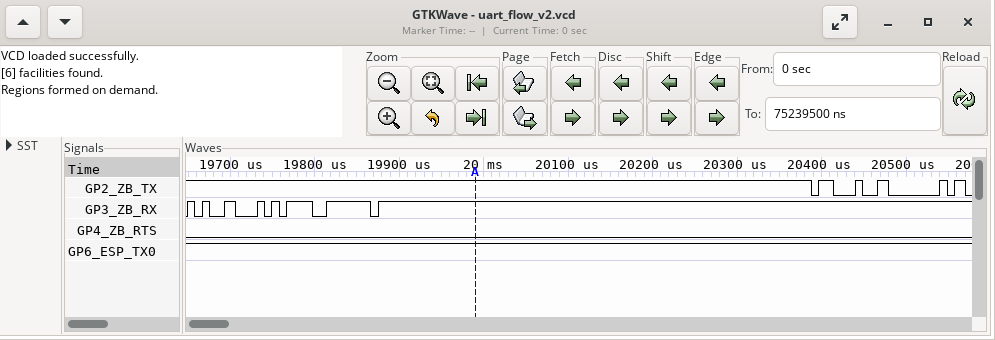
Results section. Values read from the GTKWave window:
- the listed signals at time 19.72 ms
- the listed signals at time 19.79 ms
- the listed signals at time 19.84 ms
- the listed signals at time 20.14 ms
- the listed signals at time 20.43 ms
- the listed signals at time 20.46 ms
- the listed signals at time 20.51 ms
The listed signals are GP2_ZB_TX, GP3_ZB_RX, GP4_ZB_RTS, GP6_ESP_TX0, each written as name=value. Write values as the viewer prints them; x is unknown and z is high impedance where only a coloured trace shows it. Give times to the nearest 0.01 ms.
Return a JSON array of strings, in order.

["GP2_ZB_TX=1, GP3_ZB_RX=0, GP4_ZB_RTS=0, GP6_ESP_TX0=1", "GP2_ZB_TX=1, GP3_ZB_RX=1, GP4_ZB_RTS=0, GP6_ESP_TX0=1", "GP2_ZB_TX=1, GP3_ZB_RX=1, GP4_ZB_RTS=0, GP6_ESP_TX0=1", "GP2_ZB_TX=1, GP3_ZB_RX=1, GP4_ZB_RTS=0, GP6_ESP_TX0=1", "GP2_ZB_TX=0, GP3_ZB_RX=1, GP4_ZB_RTS=0, GP6_ESP_TX0=1", "GP2_ZB_TX=0, GP3_ZB_RX=1, GP4_ZB_RTS=0, GP6_ESP_TX0=1", "GP2_ZB_TX=0, GP3_ZB_RX=1, GP4_ZB_RTS=0, GP6_ESP_TX0=1"]
